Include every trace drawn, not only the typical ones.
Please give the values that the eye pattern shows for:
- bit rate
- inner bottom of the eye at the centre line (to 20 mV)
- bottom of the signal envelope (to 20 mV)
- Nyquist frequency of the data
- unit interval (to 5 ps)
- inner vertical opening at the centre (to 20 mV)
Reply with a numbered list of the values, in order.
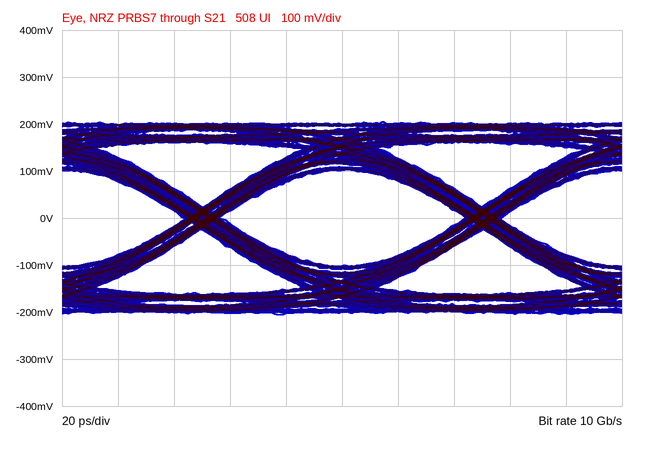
1. 10 Gb/s
2. -100 mV
3. -200 mV
4. 5 GHz
5. 100 ps
6. 200 mV
